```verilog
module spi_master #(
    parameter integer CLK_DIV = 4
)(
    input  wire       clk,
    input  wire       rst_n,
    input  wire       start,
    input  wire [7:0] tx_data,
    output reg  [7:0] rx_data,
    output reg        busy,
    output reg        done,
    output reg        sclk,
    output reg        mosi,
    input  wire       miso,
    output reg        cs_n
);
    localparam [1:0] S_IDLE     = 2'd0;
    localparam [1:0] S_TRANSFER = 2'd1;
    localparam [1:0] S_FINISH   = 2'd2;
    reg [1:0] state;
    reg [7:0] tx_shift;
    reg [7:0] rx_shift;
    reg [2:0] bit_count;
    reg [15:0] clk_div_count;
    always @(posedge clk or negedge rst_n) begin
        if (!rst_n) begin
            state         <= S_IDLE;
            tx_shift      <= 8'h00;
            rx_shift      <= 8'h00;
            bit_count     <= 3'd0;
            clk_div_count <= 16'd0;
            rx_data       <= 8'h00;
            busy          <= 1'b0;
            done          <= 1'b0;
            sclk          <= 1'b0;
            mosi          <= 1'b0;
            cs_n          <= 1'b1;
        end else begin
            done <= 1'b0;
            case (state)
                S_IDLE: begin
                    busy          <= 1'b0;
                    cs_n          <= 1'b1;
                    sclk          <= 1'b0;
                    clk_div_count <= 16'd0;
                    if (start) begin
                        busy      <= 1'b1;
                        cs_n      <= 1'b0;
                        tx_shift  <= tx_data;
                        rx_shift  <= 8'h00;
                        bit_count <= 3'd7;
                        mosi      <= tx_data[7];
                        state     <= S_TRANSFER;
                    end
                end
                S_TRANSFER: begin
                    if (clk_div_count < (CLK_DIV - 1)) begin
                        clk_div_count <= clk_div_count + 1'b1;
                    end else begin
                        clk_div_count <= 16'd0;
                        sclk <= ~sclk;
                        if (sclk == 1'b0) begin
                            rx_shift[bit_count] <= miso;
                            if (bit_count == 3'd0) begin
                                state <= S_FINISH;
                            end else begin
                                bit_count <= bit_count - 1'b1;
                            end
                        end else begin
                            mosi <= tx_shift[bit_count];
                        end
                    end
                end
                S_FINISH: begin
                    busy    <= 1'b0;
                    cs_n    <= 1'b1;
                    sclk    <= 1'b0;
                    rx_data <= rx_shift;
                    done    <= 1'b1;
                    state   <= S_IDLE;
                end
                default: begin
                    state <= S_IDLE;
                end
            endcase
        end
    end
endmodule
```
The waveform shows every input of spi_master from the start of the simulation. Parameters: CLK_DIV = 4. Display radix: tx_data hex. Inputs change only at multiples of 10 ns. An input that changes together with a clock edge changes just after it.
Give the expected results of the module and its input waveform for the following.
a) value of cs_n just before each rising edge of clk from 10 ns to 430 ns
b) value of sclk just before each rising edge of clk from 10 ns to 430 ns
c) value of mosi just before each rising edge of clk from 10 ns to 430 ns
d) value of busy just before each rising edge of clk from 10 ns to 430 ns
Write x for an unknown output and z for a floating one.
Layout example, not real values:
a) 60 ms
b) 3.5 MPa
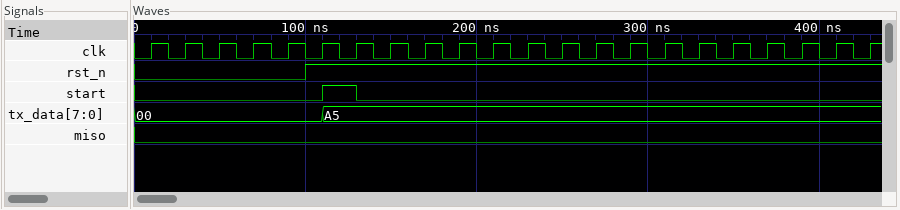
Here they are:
a) 1 1 1 1 1 1 1 0 0 0 0 0 0 0 0 0 0 0 0 0 0 0
b) 0 0 0 0 0 0 0 0 0 0 0 1 1 1 1 0 0 0 0 1 1 1
c) 0 0 0 0 0 0 0 1 1 1 1 1 1 1 1 0 0 0 0 0 0 0
d) 0 0 0 0 0 0 0 1 1 1 1 1 1 1 1 1 1 1 1 1 1 1
